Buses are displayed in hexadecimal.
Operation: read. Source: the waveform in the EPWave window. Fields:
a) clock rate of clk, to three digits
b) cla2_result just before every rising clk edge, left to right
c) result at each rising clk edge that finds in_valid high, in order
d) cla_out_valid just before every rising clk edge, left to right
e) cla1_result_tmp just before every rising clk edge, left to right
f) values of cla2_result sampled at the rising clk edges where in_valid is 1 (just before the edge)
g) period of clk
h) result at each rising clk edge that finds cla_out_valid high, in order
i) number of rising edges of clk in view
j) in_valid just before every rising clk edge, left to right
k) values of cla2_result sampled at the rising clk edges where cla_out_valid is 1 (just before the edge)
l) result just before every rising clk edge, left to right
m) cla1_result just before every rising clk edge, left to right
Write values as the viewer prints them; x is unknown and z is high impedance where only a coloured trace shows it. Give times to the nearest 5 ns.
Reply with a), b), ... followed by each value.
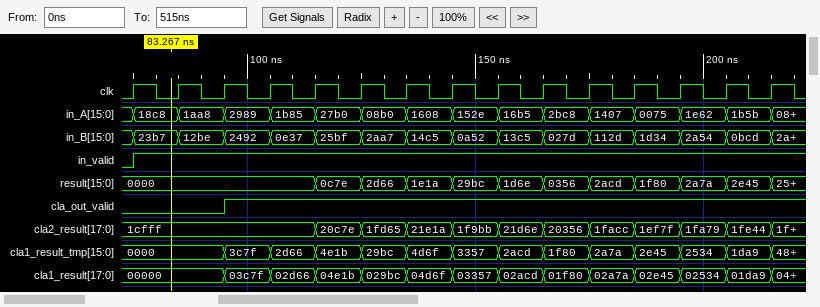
a) 100 MHz
b) 1cfff, 1cfff, 1cfff, 1cfff, 1cfff, 20c7e, 1fd65, 21e1a, 1f9bb, 21d6e, 20356, 1facc, 1ef7f, 1fa79, 1fe44
c) 0000, 0000, 0000, 0000, 0c7e, 2d66, 1e1a, 29bc, 1d6e, 0356, 2acd, 1f80, 2a7a, 2e45
d) 0 0 0 1 1 1 1 1 1 1 1 1 1 1 1
e) 0000, 0000, 0000, 3c7f, 2d66, 4e1b, 29bc, 4d6f, 3357, 2acd, 1f80, 2a7a, 2e45, 2534, 1da9
f) 1cfff, 1cfff, 1cfff, 1cfff, 20c7e, 1fd65, 21e1a, 1f9bb, 21d6e, 20356, 1facc, 1ef7f, 1fa79, 1fe44
g) 10 ns
h) 0000, 0000, 0c7e, 2d66, 1e1a, 29bc, 1d6e, 0356, 2acd, 1f80, 2a7a, 2e45
i) 15
j) 0 1 1 1 1 1 1 1 1 1 1 1 1 1 1
k) 1cfff, 1cfff, 20c7e, 1fd65, 21e1a, 1f9bb, 21d6e, 20356, 1facc, 1ef7f, 1fa79, 1fe44
l) 0000, 0000, 0000, 0000, 0000, 0c7e, 2d66, 1e1a, 29bc, 1d6e, 0356, 2acd, 1f80, 2a7a, 2e45
m) 00000, 00000, 00000, 03c7f, 02d66, 04e1b, 029bc, 04d6f, 03357, 02acd, 01f80, 02a7a, 02e45, 02534, 01da9
